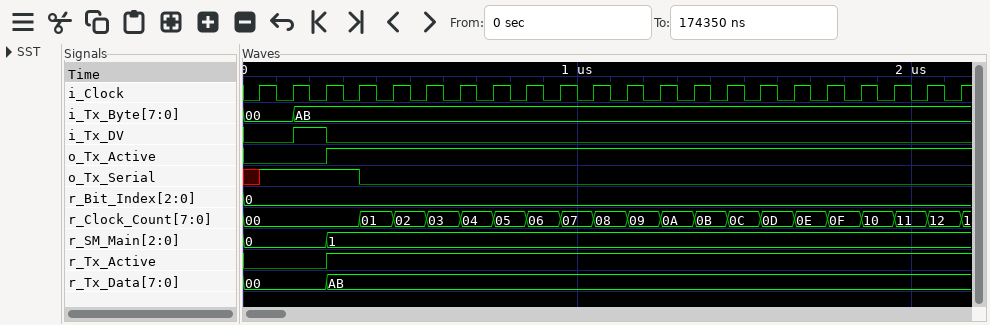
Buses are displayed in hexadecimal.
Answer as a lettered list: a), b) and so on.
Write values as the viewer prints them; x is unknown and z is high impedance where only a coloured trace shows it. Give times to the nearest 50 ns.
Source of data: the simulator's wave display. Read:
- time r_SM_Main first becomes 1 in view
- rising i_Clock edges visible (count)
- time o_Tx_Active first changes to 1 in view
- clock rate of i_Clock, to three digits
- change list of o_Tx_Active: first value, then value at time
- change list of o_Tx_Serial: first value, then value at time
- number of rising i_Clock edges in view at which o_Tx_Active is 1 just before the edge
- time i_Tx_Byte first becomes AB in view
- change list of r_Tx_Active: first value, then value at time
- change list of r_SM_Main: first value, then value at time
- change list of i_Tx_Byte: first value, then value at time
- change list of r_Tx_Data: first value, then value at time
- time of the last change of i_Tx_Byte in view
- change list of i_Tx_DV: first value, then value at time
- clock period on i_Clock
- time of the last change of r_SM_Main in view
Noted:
a) 250 ns
b) 22
c) 250 ns
d) 10.0 MHz
e) 0, 1 at 250 ns
f) x, 1 at 50 ns, 0 at 350 ns
g) 19
h) 150 ns
i) 0, 1 at 250 ns
j) 0, 1 at 250 ns
k) 00, AB at 150 ns
l) 00, AB at 250 ns
m) 150 ns
n) 0, 1 at 150 ns, 0 at 250 ns
o) 100 ns
p) 250 ns
